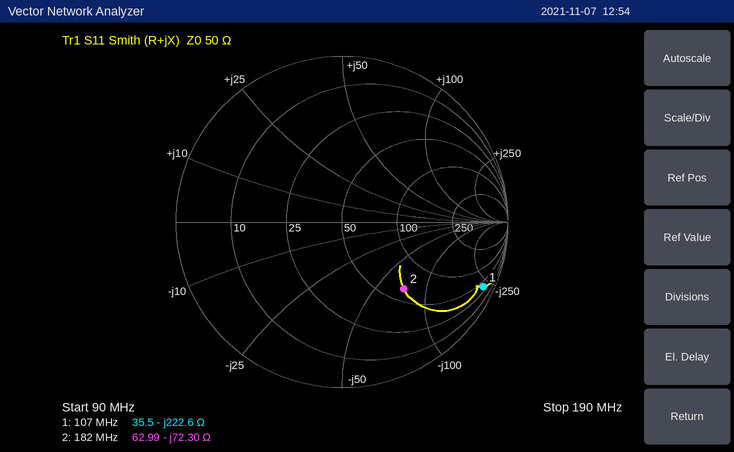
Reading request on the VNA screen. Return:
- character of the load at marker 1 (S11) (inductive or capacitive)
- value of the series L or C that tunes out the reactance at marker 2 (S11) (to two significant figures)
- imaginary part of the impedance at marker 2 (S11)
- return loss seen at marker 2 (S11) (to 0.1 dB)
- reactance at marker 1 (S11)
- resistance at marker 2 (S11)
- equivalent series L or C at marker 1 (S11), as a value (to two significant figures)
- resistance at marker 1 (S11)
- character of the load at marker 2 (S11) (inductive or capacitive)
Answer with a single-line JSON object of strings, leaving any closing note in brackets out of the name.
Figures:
{"character of the load at marker 1 (S11)": "capacitive", "value of the series L or C that tunes out the reactance at marker 2 (S11)": "63 nH", "imaginary part of the impedance at marker 2": "-72.30 Ω", "return loss seen at marker 2 (S11)": "5.2 dB", "reactance at marker 1": "-222.6 Ω", "resistance at marker 2": "62.99 Ω", "equivalent series L or C at marker 1 (S11), as a value": "6.7 pF", "resistance at marker 1": "35.5 Ω", "character of the load at marker 2 (S11)": "capacitive"}
